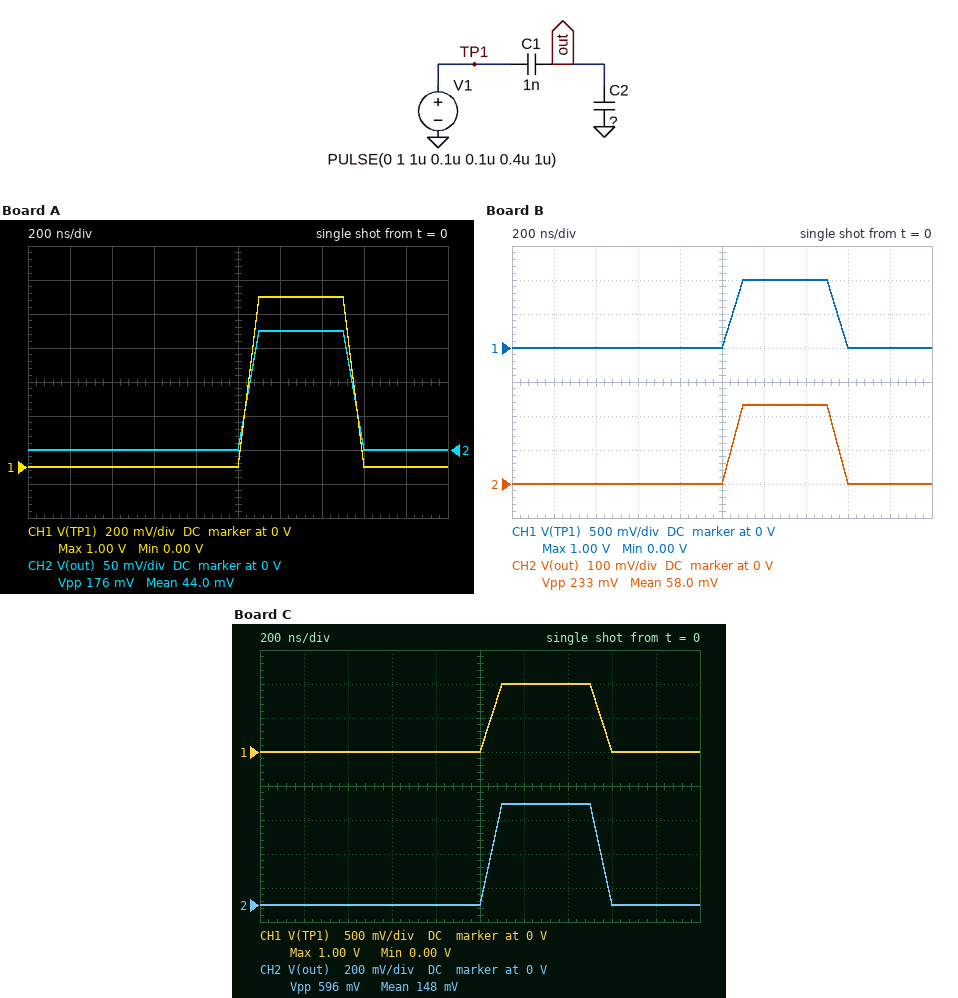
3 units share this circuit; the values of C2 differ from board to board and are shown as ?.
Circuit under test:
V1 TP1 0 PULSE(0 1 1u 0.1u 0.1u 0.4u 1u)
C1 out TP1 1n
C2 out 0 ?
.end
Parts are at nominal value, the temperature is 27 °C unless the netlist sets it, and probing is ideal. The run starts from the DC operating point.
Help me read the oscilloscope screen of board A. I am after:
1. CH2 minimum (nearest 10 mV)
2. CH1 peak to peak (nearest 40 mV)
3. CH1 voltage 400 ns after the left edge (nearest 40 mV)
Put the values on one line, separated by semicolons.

0 V; 1.00 V; 0 V
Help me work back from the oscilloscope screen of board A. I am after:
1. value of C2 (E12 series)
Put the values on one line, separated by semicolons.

4.7 nF
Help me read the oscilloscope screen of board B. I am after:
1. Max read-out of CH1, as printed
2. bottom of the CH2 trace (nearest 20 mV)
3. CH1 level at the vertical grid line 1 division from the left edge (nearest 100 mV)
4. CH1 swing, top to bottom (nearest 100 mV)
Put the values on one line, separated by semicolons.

1.00 V; 0 V; 0 V; 1.0 V
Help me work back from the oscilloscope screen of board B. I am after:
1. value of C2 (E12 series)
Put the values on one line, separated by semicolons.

3.3 nF
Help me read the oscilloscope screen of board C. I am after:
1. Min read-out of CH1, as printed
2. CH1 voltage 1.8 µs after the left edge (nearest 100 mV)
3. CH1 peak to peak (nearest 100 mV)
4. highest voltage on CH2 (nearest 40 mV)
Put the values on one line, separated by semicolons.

0.00 V; 0 V; 1.0 V; 600 mV
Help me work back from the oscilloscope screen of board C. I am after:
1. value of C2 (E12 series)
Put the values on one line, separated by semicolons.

680 pF
